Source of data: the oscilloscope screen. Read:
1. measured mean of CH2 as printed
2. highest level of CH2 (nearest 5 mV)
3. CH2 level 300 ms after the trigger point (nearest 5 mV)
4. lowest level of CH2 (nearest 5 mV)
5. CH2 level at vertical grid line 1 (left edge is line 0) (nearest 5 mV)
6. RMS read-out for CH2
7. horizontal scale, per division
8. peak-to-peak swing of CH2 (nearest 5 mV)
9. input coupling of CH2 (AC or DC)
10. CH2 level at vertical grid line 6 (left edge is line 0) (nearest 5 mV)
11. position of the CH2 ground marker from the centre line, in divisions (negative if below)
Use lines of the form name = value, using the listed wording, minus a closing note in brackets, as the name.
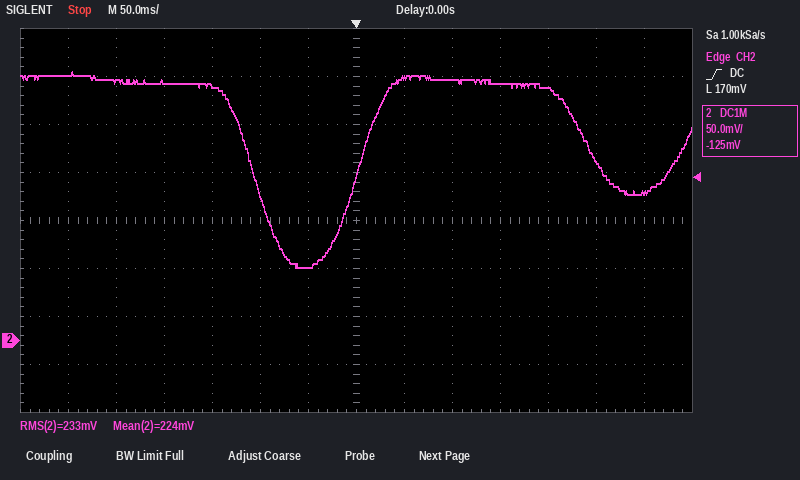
measured mean of CH2 as printed = 224 mV
highest level of CH2 = 280 mV
CH2 level 300 ms after the trigger point = 155 mV
lowest level of CH2 = 75 mV
CH2 level at vertical grid line 1 (left edge is line 0) = 275 mV
RMS read-out for CH2 = 233 mV
horizontal scale, per division = 50 ms
peak-to-peak swing of CH2 = 205 mV
input coupling of CH2 = DC
CH2 level at vertical grid line 6 (left edge is line 0) = 75 mV
position of the CH2 ground marker from the centre line, in divisions = -2.5 div
